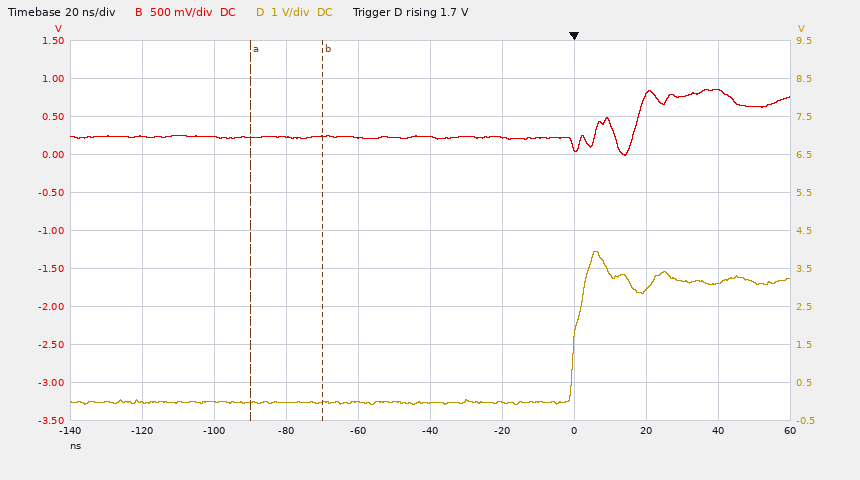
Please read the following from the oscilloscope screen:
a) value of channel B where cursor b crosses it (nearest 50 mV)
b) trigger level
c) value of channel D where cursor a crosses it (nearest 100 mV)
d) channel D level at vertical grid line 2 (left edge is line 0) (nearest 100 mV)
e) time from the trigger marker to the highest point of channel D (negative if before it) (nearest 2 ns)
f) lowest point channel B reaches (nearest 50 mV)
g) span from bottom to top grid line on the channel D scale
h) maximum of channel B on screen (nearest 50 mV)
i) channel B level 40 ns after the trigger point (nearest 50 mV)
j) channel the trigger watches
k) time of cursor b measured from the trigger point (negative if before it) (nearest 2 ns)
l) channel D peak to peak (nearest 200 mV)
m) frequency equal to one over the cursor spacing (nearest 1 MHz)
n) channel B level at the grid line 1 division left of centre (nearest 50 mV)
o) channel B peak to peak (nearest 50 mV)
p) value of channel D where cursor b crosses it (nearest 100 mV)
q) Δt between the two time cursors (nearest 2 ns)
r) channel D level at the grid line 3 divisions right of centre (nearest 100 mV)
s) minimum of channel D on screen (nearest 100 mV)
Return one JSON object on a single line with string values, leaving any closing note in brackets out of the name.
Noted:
{"value of channel B where cursor b crosses it": "250 mV", "trigger level": "1.7 V", "value of channel D where cursor a crosses it": "0.0 V", "channel D level at vertical grid line 2 (left edge is line 0)": "0.0 V", "time from the trigger marker to the highest point of channel D (negative if before it)": "+6 ns", "lowest point channel B reaches": "0 mV", "span from bottom to top grid line on the channel D scale": "10 V", "maximum of channel B on screen": "850 mV", "channel B level 40 ns after the trigger point": "850 mV", "channel the trigger watches": "channel D", "time of cursor b measured from the trigger point (negative if before it)": "-70 ns", "channel D peak to peak": "4.0 V", "frequency equal to one over the cursor spacing": "50 MHz", "channel B level at the grid line 1 division left of centre": "200 mV", "channel B peak to peak": "850 mV", "value of channel D where cursor b crosses it": "0.0 V", "Δt between the two time cursors": "20 ns", "channel D level at the grid line 3 divisions right of centre": "2.9 V", "minimum of channel D on screen": "-100 mV"}
